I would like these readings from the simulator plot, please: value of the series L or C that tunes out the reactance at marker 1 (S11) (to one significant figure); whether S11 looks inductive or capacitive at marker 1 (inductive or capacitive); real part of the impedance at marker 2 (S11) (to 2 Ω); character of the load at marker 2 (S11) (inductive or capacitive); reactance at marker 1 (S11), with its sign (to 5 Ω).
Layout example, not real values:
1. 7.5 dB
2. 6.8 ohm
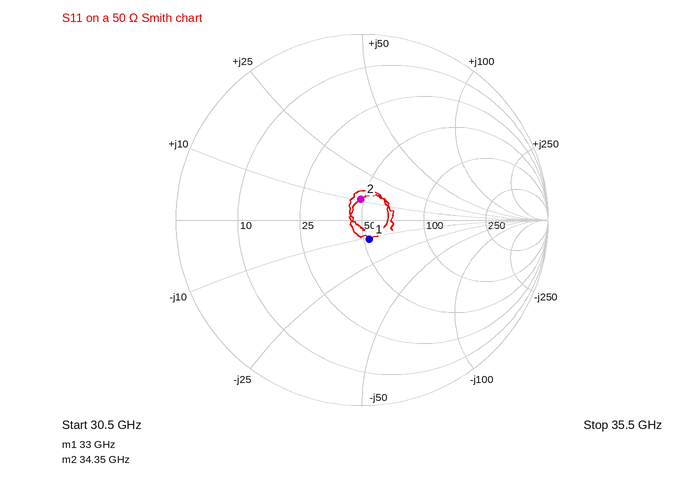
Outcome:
1. 50 pH
2. capacitive
3. 48 Ω
4. inductive
5. -10 Ω
